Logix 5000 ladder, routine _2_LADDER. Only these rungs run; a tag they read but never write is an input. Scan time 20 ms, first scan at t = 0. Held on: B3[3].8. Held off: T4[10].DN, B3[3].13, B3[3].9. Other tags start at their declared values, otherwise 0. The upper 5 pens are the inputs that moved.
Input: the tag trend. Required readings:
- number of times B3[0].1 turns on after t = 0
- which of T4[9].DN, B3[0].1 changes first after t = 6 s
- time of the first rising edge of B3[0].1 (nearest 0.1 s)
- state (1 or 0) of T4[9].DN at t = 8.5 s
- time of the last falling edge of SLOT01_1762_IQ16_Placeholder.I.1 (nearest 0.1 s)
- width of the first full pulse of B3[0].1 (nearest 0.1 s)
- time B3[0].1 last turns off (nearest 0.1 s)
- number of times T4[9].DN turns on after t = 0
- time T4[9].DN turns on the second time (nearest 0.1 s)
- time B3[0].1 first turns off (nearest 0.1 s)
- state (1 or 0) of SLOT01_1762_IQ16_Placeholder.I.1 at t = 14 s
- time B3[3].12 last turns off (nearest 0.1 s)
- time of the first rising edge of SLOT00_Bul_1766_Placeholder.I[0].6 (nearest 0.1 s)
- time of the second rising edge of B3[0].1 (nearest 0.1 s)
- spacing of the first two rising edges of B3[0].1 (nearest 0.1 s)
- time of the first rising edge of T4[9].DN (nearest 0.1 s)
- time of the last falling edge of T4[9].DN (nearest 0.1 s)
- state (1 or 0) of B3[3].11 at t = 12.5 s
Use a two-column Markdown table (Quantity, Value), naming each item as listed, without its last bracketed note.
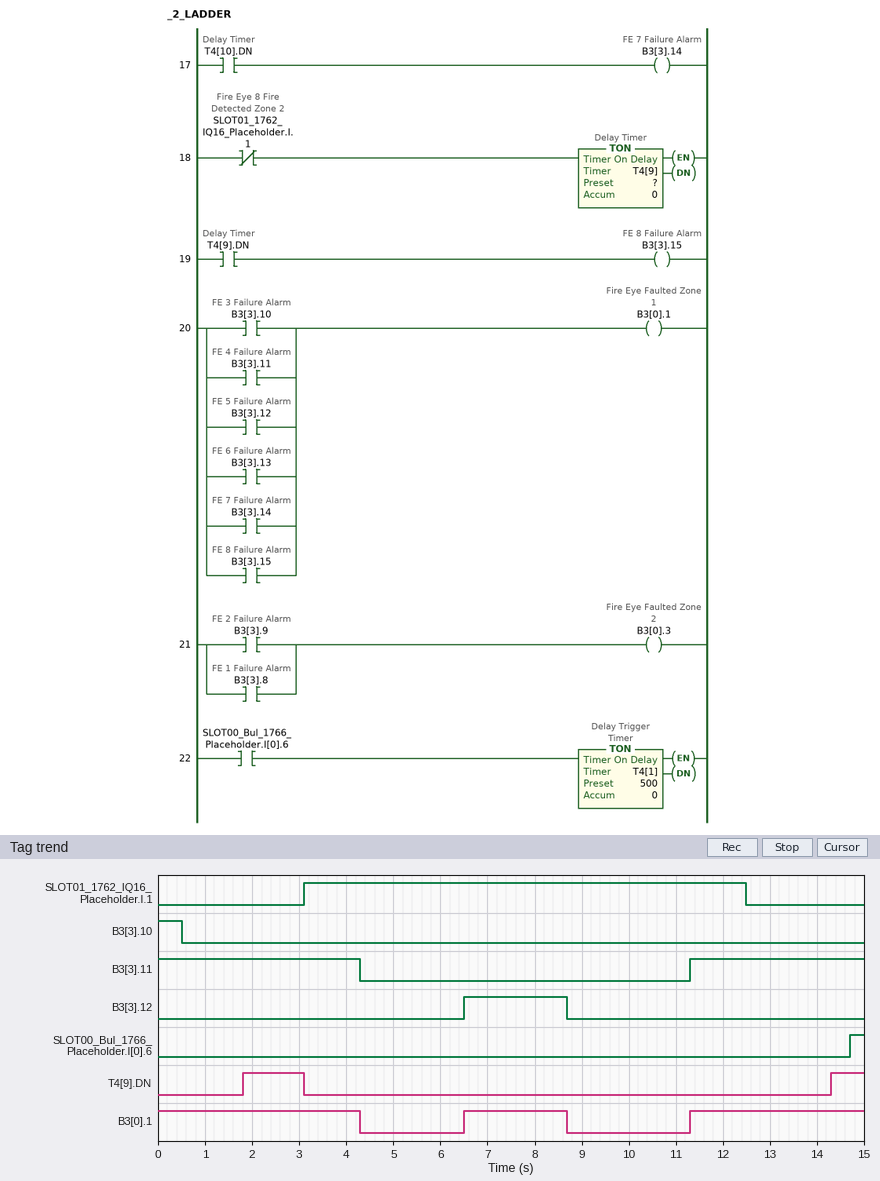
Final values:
| Quantity | Value |
|---|---|
| number of times B3[0].1 turns on after t = 0 | 2 |
| which of T4[9].DN, B3[0].1 changes first after t = 6 s | B3[0].1 |
| time of the first rising edge of B3[0].1 | 6.5 s |
| state (1 or 0) of T4[9].DN at t = 8.5 s | 0 |
| time of the last falling edge of SLOT01_1762_IQ16_Placeholder.I.1 | 12.5 s |
| width of the first full pulse of B3[0].1 | 2.2 s |
| time B3[0].1 last turns off | 8.7 s |
| number of times T4[9].DN turns on after t = 0 | 2 |
| time T4[9].DN turns on the second time | 14.3 s |
| time B3[0].1 first turns off | 4.3 s |
| state (1 or 0) of SLOT01_1762_IQ16_Placeholder.I.1 at t = 14 s | 0 |
| time B3[3].12 last turns off | 8.7 s |
| time of the first rising edge of SLOT00_Bul_1766_Placeholder.I[0].6 | 14.7 s |
| time of the second rising edge of B3[0].1 | 11.3 s |
| spacing of the first two rising edges of B3[0].1 | 4.8 s |
| time of the first rising edge of T4[9].DN | 1.8 s |
| time of the last falling edge of T4[9].DN | 3.1 s |
| state (1 or 0) of B3[3].11 at t = 12.5 s | 1 |
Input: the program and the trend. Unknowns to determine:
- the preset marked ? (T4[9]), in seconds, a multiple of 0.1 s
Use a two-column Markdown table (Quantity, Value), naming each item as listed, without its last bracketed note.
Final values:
| Quantity | Value |
|---|---|
| the preset marked ? (T4[9]), in seconds, a multiple of 0.1 s | 1.8 s |
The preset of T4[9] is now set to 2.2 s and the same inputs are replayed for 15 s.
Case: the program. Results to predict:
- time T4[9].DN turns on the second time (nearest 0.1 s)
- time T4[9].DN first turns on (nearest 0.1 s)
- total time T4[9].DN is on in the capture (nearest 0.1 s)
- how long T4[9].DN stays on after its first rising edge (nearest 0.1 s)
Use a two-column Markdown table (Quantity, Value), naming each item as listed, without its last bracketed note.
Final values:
| Quantity | Value |
|---|---|
| time T4[9].DN turns on the second time | 14.7 s |
| time T4[9].DN first turns on | 2.2 s |
| total time T4[9].DN is on in the capture | 1.2 s |
| how long T4[9].DN stays on after its first rising edge | 0.9 s |
